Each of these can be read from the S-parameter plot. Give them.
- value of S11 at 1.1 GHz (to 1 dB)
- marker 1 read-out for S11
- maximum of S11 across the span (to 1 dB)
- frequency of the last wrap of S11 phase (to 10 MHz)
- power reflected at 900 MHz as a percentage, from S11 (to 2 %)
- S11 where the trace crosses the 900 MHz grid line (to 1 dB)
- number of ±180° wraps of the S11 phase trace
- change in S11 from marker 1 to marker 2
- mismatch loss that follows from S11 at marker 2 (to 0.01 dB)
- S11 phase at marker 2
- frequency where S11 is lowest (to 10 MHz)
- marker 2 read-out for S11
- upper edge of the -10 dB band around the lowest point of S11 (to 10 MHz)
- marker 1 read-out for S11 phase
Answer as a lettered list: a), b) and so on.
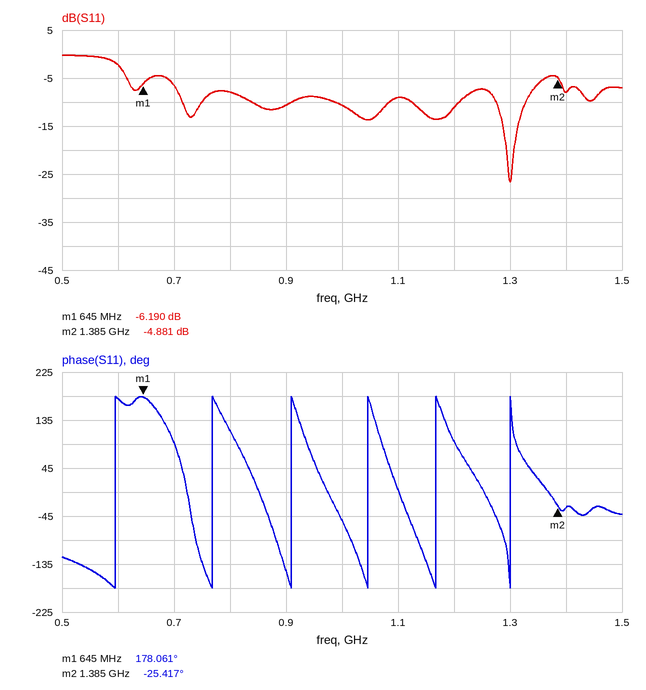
a) -9 dB
b) -6.190 dB
c) 0 dB
d) 1.30 GHz
e) 8 %
f) -11 dB
g) 6
h) 1.309 dB
i) 1.71 dB
j) -25.417°
k) 1.30 GHz
l) -4.881 dB
m) 1.33 GHz
n) 178.061°
